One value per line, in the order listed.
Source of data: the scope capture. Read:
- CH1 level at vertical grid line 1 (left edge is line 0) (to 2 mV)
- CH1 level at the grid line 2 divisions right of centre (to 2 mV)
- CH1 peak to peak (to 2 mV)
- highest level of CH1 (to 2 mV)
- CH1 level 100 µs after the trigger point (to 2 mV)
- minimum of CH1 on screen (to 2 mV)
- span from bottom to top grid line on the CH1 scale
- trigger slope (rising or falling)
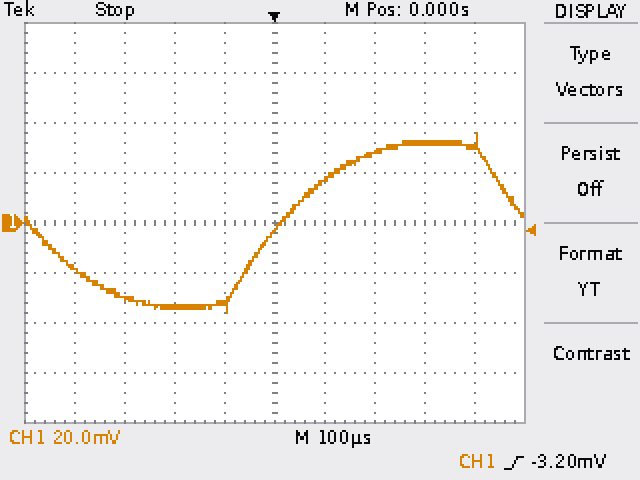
-18 mV
28 mV
72 mV
36 mV
16 mV
-36 mV
160 mV
rising
